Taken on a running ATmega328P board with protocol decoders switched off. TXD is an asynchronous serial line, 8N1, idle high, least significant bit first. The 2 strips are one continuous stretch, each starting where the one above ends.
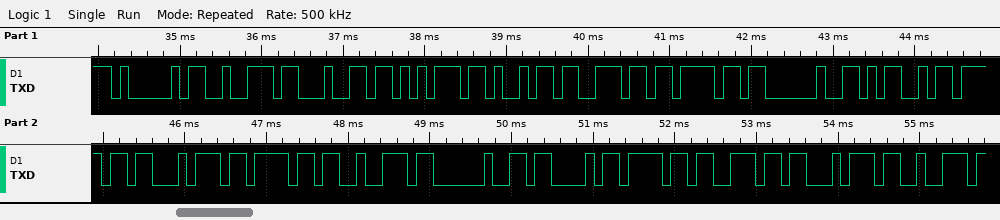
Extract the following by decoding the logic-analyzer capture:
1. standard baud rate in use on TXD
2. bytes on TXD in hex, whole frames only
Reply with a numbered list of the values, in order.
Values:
1. 9600 baud
2. 0x41 0x72 0x64 0x75 0x69 0x6E 0x6F 0x20 0x4D 0x6F 0x74 0x6F 0x72 0x20 0x43 0x6F 0x6E 0x74 0x72
